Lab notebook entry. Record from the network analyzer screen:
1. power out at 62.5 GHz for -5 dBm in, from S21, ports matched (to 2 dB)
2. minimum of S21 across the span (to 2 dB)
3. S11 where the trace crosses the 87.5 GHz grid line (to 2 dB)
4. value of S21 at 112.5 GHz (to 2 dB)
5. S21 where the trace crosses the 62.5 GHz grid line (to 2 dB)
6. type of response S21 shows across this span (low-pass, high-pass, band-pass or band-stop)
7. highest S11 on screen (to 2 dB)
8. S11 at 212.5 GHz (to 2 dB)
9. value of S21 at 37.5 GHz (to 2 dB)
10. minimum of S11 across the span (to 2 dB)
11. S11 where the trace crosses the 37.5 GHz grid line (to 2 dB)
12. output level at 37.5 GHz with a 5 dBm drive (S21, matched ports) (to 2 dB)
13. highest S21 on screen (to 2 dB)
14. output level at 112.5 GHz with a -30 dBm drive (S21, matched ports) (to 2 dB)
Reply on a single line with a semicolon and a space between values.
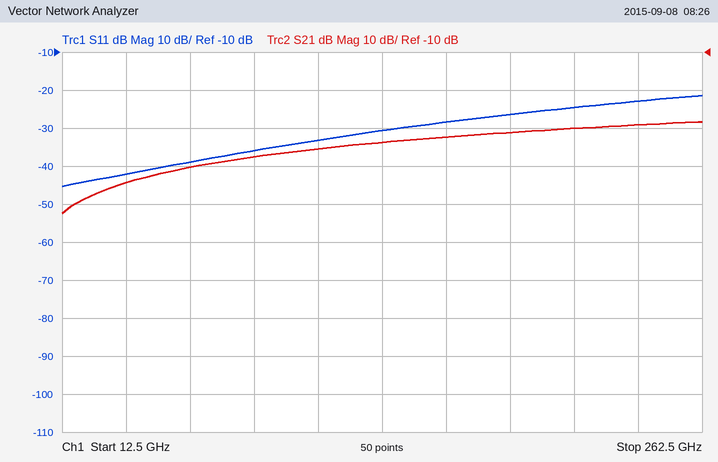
-46 dBm; -52 dB; -36 dB; -36 dB; -40 dB; high-pass; -22 dB; -24 dB; -44 dB; -46 dB; -42 dB; -40 dBm; -28 dB; -66 dBm
